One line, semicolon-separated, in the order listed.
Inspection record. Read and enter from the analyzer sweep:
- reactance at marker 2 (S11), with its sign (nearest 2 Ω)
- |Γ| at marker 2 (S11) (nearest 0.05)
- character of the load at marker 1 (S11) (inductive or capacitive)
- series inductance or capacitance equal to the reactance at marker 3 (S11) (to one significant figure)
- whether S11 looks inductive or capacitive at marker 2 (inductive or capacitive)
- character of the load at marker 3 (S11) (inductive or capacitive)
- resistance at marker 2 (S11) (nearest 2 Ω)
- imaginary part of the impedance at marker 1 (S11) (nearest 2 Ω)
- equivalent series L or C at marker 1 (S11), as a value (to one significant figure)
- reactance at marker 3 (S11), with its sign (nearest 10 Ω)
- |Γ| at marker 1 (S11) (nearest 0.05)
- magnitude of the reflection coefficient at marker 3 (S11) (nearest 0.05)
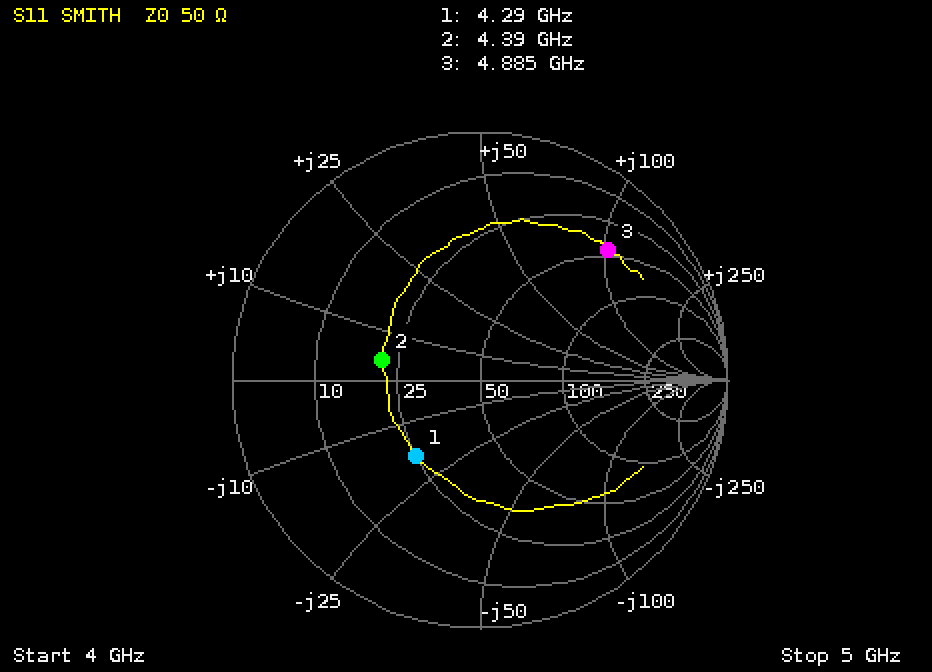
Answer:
+4 Ω; 0.40; capacitive; 3 nH; inductive; inductive; 22 Ω; -18 Ω; 2 pF; +100 Ω; 0.40; 0.75
